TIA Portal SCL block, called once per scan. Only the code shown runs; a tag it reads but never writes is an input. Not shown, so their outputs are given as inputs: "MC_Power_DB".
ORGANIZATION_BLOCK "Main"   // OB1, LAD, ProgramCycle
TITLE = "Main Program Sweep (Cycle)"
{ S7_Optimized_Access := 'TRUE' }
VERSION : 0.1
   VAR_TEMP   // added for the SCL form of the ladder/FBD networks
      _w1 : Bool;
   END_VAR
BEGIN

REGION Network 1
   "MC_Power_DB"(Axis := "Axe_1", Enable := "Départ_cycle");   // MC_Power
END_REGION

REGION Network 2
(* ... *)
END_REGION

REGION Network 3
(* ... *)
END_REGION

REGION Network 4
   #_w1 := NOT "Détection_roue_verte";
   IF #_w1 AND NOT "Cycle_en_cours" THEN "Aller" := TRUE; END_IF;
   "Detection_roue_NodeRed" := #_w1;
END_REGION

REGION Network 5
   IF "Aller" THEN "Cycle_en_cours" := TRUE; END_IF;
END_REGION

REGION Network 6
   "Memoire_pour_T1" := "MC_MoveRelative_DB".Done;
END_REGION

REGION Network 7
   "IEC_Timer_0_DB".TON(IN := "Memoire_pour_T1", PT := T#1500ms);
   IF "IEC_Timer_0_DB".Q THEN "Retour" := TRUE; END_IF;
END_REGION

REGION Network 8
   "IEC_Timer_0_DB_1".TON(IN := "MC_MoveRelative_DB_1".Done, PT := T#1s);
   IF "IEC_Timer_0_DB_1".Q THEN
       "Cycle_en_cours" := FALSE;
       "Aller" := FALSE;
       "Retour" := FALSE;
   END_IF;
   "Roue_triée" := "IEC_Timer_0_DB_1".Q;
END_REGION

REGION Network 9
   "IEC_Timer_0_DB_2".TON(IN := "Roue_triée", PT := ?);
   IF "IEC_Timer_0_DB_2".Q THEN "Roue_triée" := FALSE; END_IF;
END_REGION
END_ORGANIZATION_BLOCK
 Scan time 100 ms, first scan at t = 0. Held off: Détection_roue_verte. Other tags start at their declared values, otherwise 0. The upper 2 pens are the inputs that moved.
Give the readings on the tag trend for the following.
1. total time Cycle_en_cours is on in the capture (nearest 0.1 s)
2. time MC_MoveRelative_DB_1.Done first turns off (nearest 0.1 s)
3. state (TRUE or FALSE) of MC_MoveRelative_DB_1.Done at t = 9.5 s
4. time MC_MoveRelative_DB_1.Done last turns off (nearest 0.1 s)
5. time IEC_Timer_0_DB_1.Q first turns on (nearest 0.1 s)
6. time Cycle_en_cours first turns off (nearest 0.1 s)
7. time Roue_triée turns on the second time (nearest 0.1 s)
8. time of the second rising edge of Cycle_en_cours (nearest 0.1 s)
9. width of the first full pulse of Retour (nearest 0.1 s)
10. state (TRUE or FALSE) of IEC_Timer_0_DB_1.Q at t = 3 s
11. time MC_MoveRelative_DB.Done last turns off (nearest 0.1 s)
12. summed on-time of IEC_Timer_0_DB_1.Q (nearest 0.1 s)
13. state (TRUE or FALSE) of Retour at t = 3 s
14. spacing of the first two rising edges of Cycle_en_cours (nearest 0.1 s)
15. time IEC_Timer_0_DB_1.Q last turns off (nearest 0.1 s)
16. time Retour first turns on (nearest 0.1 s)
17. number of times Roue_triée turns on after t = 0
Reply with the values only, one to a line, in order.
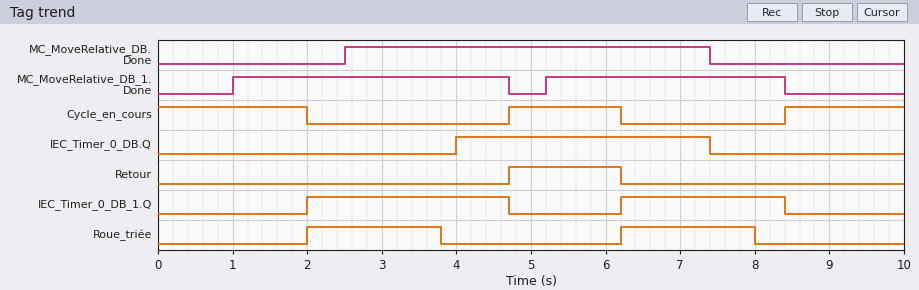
5.1 s
4.7 s
FALSE
8.4 s
2.0 s
2.0 s
6.2 s
8.4 s
1.5 s
TRUE
7.4 s
4.9 s
FALSE
3.7 s
8.4 s
4.7 s
2
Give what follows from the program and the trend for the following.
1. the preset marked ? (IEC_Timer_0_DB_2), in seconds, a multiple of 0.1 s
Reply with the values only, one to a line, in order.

1.8 s
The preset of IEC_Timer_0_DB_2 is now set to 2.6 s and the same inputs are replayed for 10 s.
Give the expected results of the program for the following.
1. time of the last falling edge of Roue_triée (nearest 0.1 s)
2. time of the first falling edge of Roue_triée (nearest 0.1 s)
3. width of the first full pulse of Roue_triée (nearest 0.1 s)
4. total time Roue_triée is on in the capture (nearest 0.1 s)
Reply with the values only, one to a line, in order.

8.4 s
4.6 s
2.6 s
4.8 s
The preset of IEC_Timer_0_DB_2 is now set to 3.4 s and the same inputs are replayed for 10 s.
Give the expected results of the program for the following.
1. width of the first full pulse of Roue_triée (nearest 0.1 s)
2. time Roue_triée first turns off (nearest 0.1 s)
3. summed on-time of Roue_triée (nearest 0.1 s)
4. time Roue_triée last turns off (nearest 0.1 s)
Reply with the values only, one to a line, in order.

2.7 s
4.7 s
4.9 s
8.4 s
